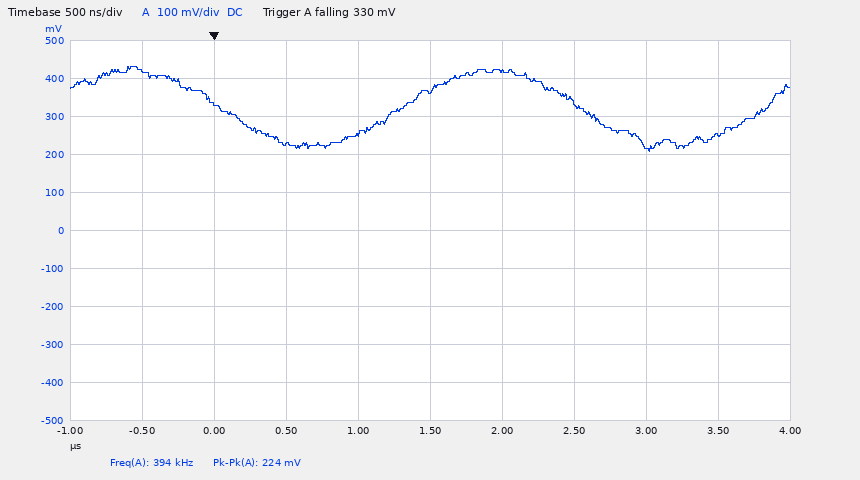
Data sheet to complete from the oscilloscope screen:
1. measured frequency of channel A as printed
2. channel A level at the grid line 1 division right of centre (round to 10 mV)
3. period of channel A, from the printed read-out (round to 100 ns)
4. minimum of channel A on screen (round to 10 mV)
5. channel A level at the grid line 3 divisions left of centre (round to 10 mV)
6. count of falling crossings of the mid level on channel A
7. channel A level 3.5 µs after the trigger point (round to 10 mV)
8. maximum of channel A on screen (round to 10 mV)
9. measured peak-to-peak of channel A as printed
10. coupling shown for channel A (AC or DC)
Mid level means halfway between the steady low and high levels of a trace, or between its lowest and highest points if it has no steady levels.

394 kHz
420 mV
2.5 µs
210 mV
330 mV
2
250 mV
430 mV
224 mV
DC
